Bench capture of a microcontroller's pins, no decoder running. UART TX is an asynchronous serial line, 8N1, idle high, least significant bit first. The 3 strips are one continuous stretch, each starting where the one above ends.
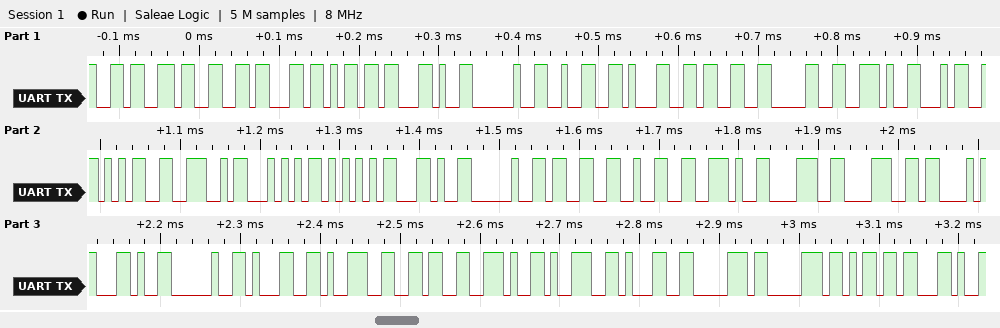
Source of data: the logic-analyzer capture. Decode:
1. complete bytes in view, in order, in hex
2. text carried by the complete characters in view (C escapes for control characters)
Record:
36 33 63 6D 2C 20 32 31 33 30 2E 34 35 4E 54 55 2C 20 33 32 2E 38 38 43 2C 20 31 39 36 2E 39 31 70 70 6D 2C
"63cm, 2130.45NTU, 32.88C, 196.91ppm,"
